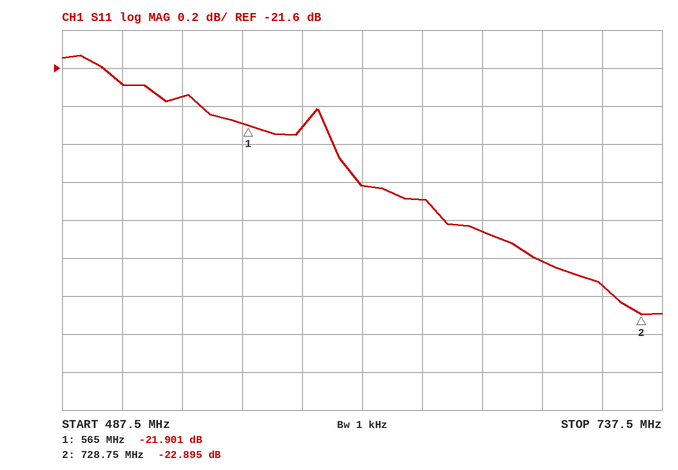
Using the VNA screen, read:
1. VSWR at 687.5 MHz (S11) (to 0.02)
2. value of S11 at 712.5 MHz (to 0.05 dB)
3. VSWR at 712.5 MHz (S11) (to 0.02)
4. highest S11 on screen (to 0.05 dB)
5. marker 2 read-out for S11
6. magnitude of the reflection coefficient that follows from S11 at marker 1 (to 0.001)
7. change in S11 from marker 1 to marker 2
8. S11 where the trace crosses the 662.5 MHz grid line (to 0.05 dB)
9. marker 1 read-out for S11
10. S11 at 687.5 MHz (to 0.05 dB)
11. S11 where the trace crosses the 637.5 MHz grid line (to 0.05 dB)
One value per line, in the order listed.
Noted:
1.16
-22.75 dB
1.16
-21.55 dB
-22.895 dB
0.080
-0.994 dB
-22.45 dB
-21.901 dB
-22.60 dB
-22.30 dB
